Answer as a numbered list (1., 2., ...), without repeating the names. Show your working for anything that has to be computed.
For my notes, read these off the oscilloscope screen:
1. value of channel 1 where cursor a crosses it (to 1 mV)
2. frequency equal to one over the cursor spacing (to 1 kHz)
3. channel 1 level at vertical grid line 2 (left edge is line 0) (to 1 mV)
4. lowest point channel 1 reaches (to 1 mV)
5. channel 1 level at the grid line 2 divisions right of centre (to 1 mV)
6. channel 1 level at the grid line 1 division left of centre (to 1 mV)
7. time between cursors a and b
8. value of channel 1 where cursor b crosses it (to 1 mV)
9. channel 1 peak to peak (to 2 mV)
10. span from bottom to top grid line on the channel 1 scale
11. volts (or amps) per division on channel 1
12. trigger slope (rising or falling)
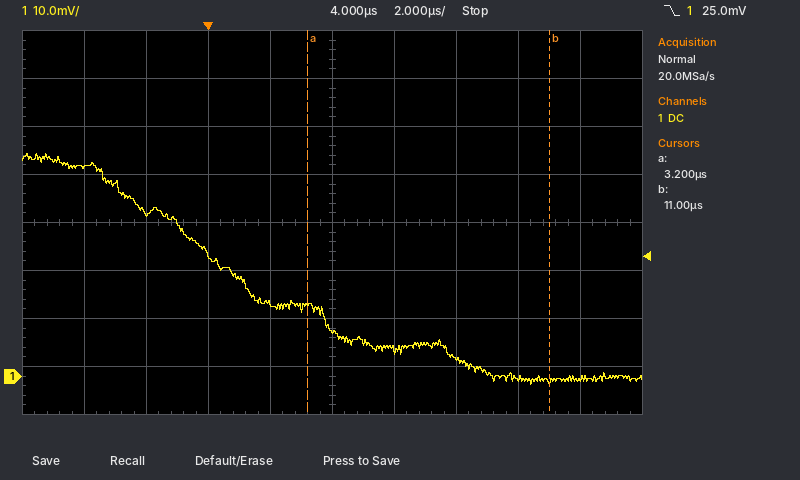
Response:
1. 15 mV
2. 1 / 7.8 µs ≈ 128 kHz
3. 34 mV
4. -2 mV
5. 4 mV
6. 15 mV
7. 11 µs − (3.2 µs) = 7.8 µs
8. -1 mV
9. 48 mV
10. 80 mV
11. 10 mV
12. falling
